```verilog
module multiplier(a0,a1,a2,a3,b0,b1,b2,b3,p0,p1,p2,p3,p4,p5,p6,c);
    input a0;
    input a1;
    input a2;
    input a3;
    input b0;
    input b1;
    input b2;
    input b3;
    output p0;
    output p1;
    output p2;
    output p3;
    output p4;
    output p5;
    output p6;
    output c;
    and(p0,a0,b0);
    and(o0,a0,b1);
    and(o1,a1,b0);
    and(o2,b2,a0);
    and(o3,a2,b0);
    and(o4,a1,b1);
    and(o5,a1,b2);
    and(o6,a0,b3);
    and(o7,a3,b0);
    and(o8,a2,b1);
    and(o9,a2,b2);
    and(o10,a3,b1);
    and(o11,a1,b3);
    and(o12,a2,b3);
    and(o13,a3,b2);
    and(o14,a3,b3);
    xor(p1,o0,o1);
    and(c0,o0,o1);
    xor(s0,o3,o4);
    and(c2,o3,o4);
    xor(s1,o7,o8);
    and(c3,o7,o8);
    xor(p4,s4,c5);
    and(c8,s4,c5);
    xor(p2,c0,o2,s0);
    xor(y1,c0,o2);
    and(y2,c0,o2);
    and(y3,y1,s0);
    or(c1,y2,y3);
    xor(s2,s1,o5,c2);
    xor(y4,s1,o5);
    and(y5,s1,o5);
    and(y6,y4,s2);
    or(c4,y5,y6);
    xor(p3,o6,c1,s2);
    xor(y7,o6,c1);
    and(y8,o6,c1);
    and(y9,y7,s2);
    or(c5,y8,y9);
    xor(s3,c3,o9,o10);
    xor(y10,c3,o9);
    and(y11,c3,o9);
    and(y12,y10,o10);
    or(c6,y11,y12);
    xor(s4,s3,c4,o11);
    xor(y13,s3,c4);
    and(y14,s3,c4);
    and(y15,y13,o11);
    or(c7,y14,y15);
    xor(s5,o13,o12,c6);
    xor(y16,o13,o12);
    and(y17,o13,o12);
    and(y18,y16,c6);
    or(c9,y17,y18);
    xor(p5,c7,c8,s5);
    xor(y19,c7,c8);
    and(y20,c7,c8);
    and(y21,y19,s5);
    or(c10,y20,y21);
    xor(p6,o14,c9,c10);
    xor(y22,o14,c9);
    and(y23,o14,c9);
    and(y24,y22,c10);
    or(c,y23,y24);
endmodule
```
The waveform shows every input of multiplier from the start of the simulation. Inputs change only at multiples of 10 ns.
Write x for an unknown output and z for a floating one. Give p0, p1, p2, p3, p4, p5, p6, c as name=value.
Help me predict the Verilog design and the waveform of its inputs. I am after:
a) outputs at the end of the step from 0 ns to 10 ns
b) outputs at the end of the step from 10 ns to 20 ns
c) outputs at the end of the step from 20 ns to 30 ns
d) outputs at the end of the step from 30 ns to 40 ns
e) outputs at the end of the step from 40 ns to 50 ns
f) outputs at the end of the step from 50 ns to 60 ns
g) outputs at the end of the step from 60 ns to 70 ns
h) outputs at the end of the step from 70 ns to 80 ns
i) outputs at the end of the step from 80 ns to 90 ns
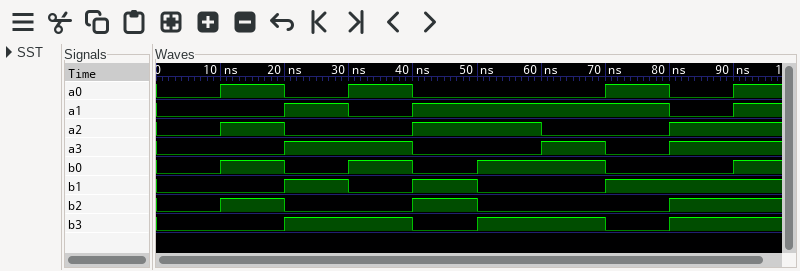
p0=0, p1=0, p2=0, p3=0, p4=0, p5=0, p6=0, c=0
p0=1, p1=0, p2=0, p3=1, p4=1, p5=0, p6=0, c=0
p0=0, p1=0, p2=1, p3=0, p4=0, p5=1, p6=1, c=0
p0=1, p1=0, p2=0, p3=0, p4=0, p5=1, p6=1, c=0
p0=0, p1=0, p2=1, p3=0, p4=0, p5=1, p6=0, c=0
p0=0, p1=1, p2=1, p3=0, p4=1, p5=1, p6=0, c=0
p0=0, p1=1, p2=0, p3=1, p4=0, p5=1, p6=1, c=0
p0=0, p1=1, p2=1, p3=0, p4=0, p5=0, p6=0, c=0
p0=0, p1=0, p2=0, p3=1, p4=1, p5=1, p6=0, c=1
